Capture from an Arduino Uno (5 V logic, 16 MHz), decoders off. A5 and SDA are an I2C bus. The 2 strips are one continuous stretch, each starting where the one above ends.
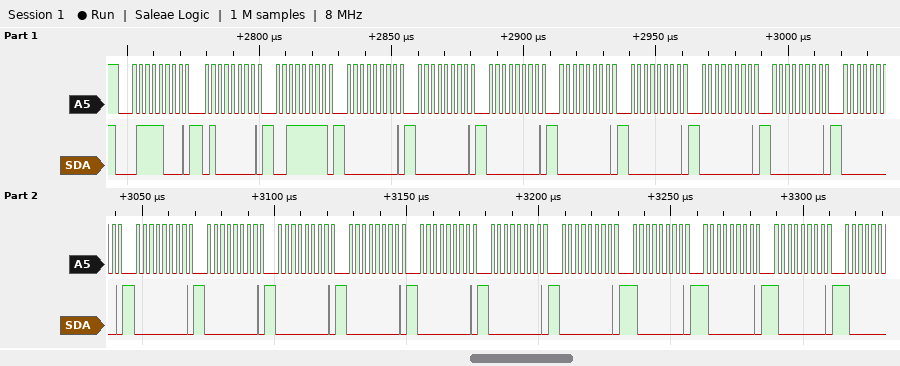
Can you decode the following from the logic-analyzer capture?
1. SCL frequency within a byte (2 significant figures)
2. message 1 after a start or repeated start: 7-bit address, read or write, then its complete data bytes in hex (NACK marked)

400 kHz
0x3C write: 40 3F 00 00 00 00 00 00 00 00 00 00 00 00 00 00 00 80 80 80
